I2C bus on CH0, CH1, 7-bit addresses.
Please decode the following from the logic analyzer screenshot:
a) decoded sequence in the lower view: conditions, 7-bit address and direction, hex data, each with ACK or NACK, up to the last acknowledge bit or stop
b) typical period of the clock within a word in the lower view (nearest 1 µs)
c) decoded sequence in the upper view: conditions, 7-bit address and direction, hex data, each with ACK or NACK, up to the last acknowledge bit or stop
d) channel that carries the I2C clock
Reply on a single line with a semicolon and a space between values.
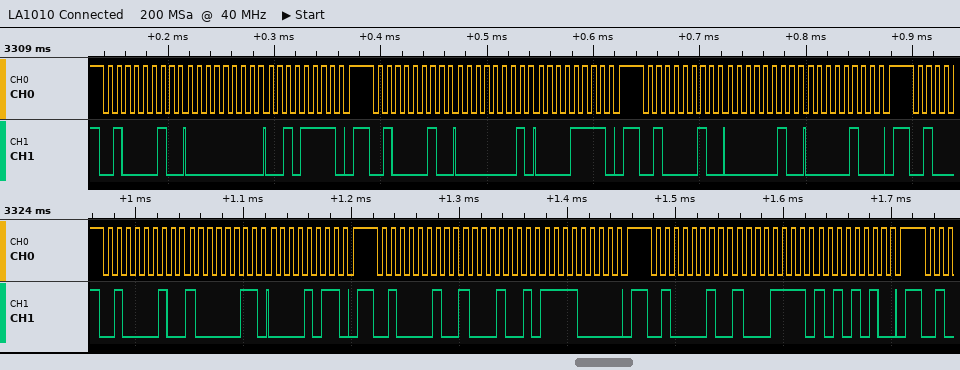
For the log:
start, address 21 write ACK, 83 ACK, 0B ACK, stop, start, address 21 write ACK, 89 ACK, F0 ACK, stop, start, address 21 write ACK, 8F ACK, AA ACK, stop; 8 µs; start, address 21 write ACK, 00 ACK, 2F ACK, stop, start, address 21 write ACK, 01 ACK, 0F ACK, stop, start, address 21 write ACK, 02 ACK, 04 ACK, stop; CH0
